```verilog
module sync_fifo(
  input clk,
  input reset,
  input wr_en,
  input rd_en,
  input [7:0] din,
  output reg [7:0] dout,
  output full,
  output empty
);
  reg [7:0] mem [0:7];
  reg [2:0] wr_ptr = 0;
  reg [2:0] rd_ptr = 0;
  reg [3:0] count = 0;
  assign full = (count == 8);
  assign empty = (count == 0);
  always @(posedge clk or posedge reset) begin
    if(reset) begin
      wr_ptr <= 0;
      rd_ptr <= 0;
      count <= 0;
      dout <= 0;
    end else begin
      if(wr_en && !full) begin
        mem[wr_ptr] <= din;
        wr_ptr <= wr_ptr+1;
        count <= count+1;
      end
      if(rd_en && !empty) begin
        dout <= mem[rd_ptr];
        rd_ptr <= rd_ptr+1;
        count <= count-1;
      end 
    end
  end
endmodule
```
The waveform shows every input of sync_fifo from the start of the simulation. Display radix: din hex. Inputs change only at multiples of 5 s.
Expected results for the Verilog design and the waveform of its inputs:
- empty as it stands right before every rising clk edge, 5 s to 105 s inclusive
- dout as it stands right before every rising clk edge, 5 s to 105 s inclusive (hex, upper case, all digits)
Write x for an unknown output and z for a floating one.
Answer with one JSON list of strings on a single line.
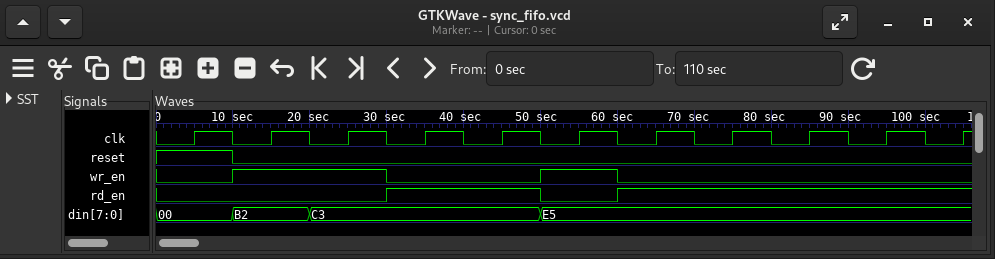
["1 1 0 0 0 1 0 1 1 1 1", "00, 00, 00, 00, B2, C3, C3, E5, E5, E5, E5"]
